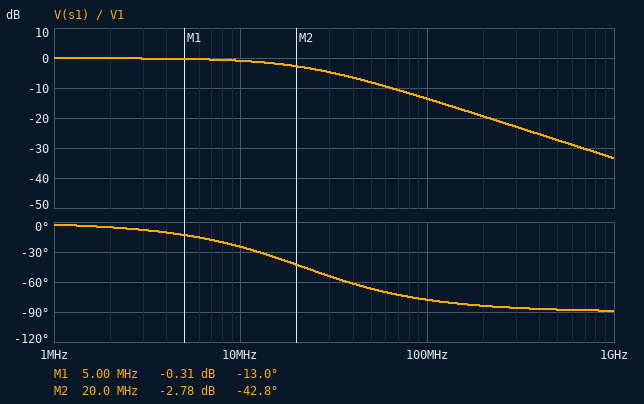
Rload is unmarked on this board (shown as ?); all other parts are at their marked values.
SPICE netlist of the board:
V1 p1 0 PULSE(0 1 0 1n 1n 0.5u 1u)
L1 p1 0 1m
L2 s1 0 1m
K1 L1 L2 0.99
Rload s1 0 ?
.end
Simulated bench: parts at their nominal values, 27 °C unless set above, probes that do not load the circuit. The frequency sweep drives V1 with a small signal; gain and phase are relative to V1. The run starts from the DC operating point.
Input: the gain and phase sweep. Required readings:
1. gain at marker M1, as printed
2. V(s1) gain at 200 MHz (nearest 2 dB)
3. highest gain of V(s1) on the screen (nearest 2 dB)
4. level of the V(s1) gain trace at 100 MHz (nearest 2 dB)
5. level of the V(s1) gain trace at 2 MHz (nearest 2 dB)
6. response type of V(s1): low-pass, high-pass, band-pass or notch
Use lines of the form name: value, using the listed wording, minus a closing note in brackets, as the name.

gain at marker M1, as printed: -0.31 dB
V(s1) gain at 200 MHz: -20 dB
highest gain of V(s1) on the screen: 0 dB
level of the V(s1) gain trace at 100 MHz: -14 dB
level of the V(s1) gain trace at 2 MHz: 0 dB
response type of V(s1): low-pass, high-pass, band-pass or notch: low-pass
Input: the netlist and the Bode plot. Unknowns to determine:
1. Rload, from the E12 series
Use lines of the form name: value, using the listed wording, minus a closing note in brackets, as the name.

Rload, from the E12 series: 2.7 kΩ
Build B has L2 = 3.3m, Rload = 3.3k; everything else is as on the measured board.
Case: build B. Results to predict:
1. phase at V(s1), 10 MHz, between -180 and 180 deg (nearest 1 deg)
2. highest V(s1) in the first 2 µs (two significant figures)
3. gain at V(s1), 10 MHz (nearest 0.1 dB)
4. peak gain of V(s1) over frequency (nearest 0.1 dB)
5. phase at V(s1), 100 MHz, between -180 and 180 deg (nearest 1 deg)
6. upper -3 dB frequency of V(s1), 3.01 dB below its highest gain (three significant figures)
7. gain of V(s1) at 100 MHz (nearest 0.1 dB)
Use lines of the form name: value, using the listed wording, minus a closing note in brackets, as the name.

phase at V(s1), 10 MHz, between -180 and 180 deg: -51 deg
highest V(s1) in the first 2 µs: 1.8 V
gain at V(s1), 10 MHz: 1.0 dB
peak gain of V(s1) over frequency: 5.1 dB
phase at V(s1), 100 MHz, between -180 and 180 deg: -85 deg
upper -3 dB frequency of V(s1), 3.01 dB below its highest gain: 8.00 MHz
gain of V(s1) at 100 MHz: -16.9 dB
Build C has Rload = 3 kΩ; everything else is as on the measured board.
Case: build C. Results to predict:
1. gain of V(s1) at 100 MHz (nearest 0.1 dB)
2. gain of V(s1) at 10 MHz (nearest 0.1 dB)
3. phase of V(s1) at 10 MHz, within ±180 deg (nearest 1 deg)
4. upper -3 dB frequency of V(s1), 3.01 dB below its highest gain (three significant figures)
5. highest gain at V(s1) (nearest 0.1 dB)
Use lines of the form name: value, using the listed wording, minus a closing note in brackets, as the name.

gain of V(s1) at 100 MHz: -12.7 dB
gain of V(s1) at 10 MHz: -0.8 dB
phase of V(s1) at 10 MHz, within ±180 deg: -23 deg
upper -3 dB frequency of V(s1), 3.01 dB below its highest gain: 24.0 MHz
highest gain at V(s1): -0.1 dB
